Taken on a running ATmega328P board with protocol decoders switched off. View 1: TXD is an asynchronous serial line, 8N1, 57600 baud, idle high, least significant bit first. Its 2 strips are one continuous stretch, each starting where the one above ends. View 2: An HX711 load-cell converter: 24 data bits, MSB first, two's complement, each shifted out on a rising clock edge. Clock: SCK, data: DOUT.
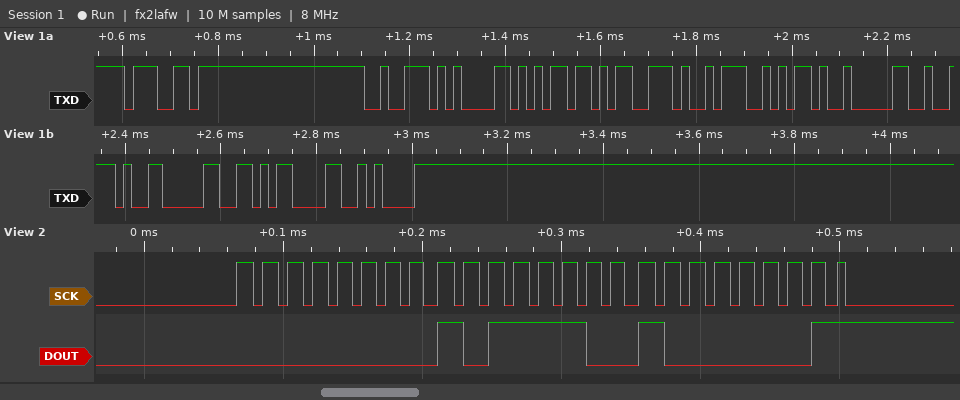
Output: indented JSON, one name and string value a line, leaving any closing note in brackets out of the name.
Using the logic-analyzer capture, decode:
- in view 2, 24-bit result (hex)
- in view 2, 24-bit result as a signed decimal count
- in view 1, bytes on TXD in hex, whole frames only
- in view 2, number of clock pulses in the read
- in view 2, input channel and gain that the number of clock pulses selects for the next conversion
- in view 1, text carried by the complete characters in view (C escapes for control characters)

{
  "in view 2, 24-bit result": "0x00BC81",
  "in view 2, 24-bit result as a signed decimal count": "48257",
  "in view 1, bytes on TXD in hex, whole frames only": "67 72 61 6D 73 3A 2D 30 2E 30 0D 0A",
  "in view 2, number of clock pulses in the read": "25",
  "in view 2, input channel and gain that the number of clock pulses selects for the next conversion": "channel A, gain 128",
  "in view 1, text carried by the complete characters in view": "\"grams:-0.0\\r\\n\""
}
